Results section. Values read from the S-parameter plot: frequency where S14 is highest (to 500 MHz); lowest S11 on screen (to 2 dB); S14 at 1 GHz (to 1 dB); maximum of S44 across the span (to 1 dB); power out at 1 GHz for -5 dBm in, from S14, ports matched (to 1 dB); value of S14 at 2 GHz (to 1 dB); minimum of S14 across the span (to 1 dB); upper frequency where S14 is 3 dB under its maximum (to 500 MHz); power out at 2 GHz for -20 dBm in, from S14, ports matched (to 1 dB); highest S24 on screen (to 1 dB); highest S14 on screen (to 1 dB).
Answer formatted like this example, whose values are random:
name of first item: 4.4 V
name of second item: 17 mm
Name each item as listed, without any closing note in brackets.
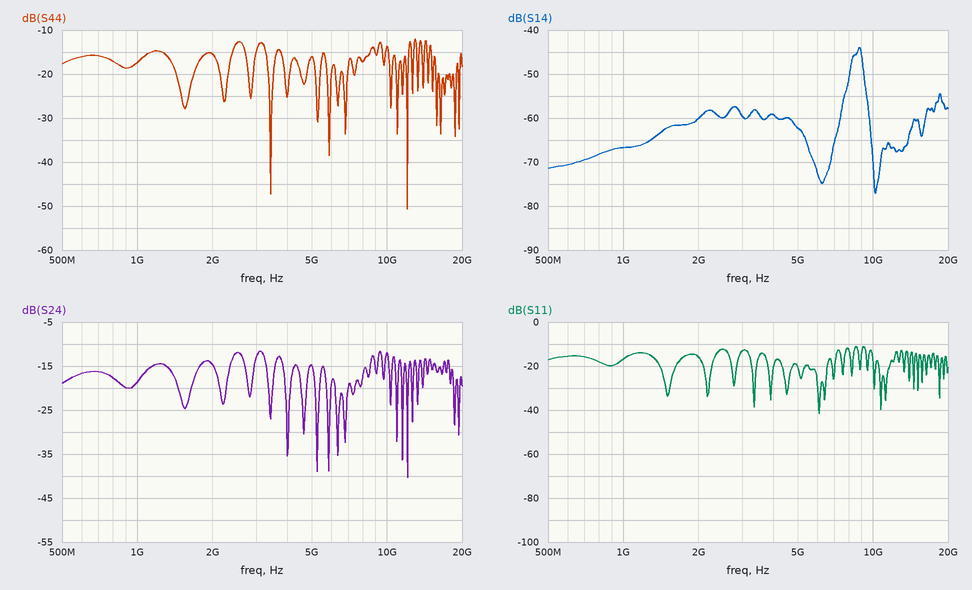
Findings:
frequency where S14 is highest: 9.0 GHz
lowest S11 on screen: -42 dB
S14 at 1 GHz: -67 dB
maximum of S44 across the span: -12 dB
power out at 1 GHz for -5 dBm in, from S14, ports matched: -72 dBm
value of S14 at 2 GHz: -60 dB
minimum of S14 across the span: -77 dB
upper frequency where S14 is 3 dB under its maximum: 9.0 GHz
power out at 2 GHz for -20 dBm in, from S14, ports matched: -80 dBm
highest S24 on screen: -12 dB
highest S14 on screen: -44 dB
